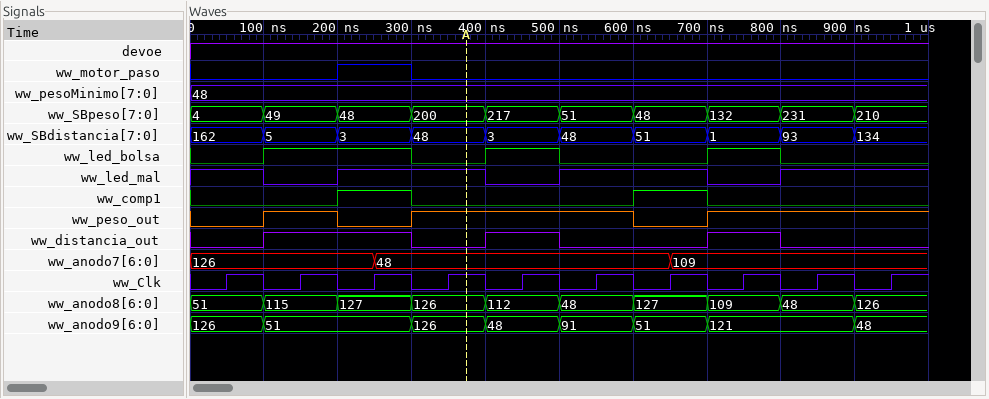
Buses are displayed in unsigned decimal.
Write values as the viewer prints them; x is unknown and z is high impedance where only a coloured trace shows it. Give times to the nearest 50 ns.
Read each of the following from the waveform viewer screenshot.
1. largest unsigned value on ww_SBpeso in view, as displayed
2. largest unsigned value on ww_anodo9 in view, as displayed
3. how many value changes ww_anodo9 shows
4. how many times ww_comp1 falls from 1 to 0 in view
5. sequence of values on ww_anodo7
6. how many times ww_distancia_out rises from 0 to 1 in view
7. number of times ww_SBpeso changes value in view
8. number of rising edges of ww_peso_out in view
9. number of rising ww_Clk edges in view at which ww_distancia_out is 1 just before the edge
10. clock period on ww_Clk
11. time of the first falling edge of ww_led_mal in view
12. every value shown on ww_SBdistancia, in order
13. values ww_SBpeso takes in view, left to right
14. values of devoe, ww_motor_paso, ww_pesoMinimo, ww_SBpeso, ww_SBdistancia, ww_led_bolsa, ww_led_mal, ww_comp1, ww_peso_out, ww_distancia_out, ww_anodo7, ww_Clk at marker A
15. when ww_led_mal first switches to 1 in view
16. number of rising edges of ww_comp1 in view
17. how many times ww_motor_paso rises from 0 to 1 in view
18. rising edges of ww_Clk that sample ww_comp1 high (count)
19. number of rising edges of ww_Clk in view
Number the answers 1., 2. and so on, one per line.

1. 231
2. 126
3. 7
4. 2
5. 126, 48, 109
6. 3
7. 9
8. 3
9. 4
10. 100 ns
11. 100 ns
12. 162, 5, 3, 48, 3, 48, 51, 1, 93, 134
13. 4, 49, 48, 200, 217, 51, 48, 132, 231, 210
14. devoe=1, ww_motor_paso=0, ww_pesoMinimo=48, ww_SBpeso=200, ww_SBdistancia=48, ww_led_bolsa=0, ww_led_mal=1, ww_comp1=0, ww_peso_out=1, ww_distancia_out=0, ww_anodo7=48, ww_Clk=1
15. 200 ns
16. 2
17. 1
18. 2
19. 10
